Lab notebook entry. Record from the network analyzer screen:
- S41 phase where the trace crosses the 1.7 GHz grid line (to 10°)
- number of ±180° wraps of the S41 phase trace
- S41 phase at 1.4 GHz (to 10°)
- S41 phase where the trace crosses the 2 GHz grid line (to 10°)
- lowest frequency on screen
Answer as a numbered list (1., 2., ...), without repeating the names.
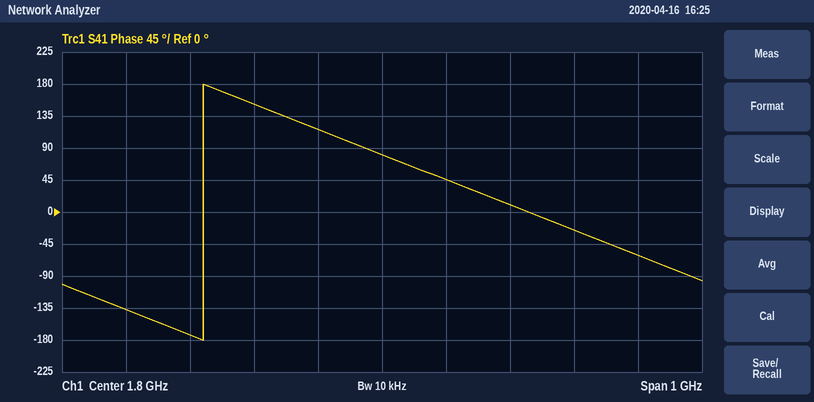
1. 120°
2. 1
3. -140°
4. 10°
5. 1.3 GHz
